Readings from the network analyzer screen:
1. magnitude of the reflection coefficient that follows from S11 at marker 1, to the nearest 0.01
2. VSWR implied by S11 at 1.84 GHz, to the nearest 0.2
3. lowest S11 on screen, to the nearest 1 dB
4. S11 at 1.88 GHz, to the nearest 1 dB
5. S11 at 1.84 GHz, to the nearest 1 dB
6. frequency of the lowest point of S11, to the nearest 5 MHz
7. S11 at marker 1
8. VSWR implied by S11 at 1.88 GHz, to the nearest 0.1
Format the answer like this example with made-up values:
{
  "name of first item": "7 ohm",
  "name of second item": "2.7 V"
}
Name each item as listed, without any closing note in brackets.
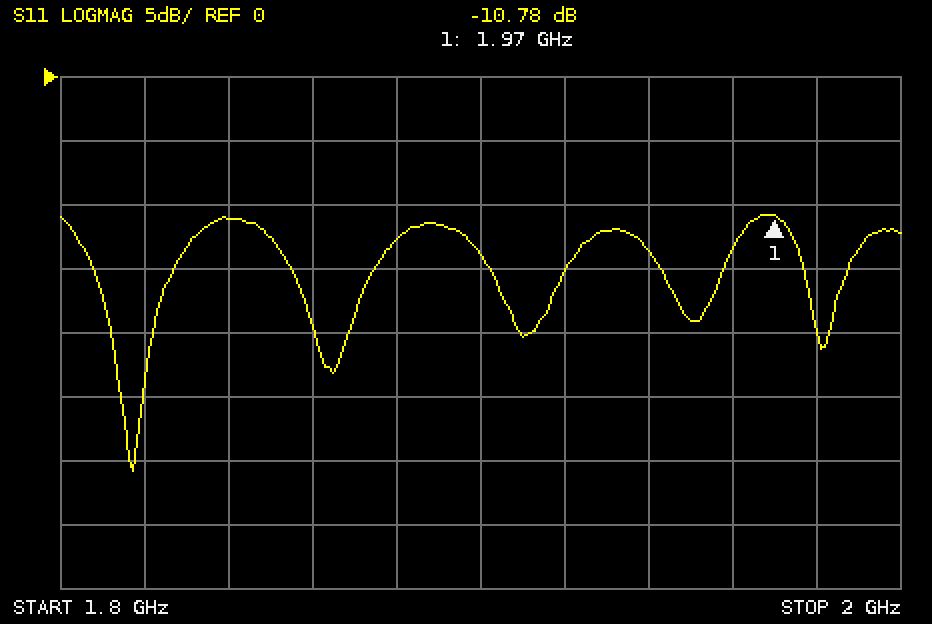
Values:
{
  "magnitude of the reflection coefficient that follows from S11 at marker 1, to the nearest 0.01": "0.29",
  "VSWR implied by S11 at 1.84 GHz, to the nearest 0.2": "1.8",
  "lowest S11 on screen, to the nearest 1 dB": "-31 dB",
  "S11 at 1.88 GHz, to the nearest 1 dB": "-13 dB",
  "S11 at 1.84 GHz, to the nearest 1 dB": "-11 dB",
  "frequency of the lowest point of S11, to the nearest 5 MHz": "1.815 GHz",
  "S11 at marker 1": "-10.78 dB",
  "VSWR implied by S11 at 1.88 GHz, to the nearest 0.1": "1.6"
}
